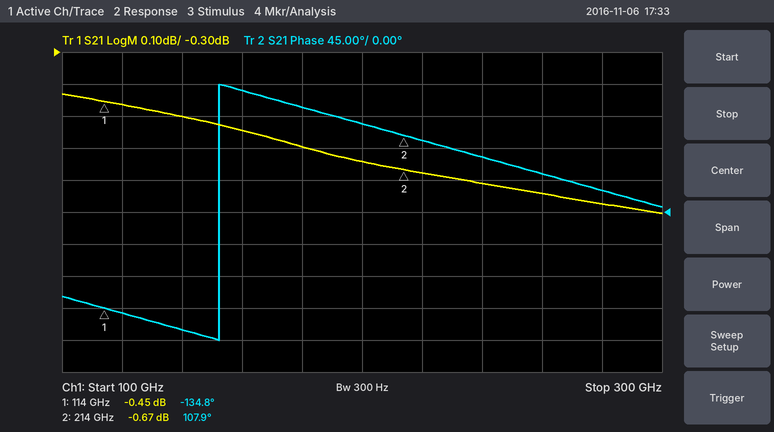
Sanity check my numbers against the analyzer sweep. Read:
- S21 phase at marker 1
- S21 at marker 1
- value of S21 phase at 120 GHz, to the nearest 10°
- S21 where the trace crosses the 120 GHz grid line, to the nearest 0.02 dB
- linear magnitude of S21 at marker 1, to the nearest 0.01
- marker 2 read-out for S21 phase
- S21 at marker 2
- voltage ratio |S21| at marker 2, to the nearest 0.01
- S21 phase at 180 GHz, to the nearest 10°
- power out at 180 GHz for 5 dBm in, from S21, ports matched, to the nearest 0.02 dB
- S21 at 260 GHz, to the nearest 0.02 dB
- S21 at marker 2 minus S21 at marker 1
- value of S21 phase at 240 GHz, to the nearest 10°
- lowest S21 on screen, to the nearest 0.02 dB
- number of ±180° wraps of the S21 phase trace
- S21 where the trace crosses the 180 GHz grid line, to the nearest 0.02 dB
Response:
-134.8°
-0.45 dB
-140°
-0.46 dB
0.95
107.9°
-0.67 dB
0.93
150°
4.40 dBm
-0.74 dB
-0.22 dB
80°
-0.80 dB
1
-0.60 dB
